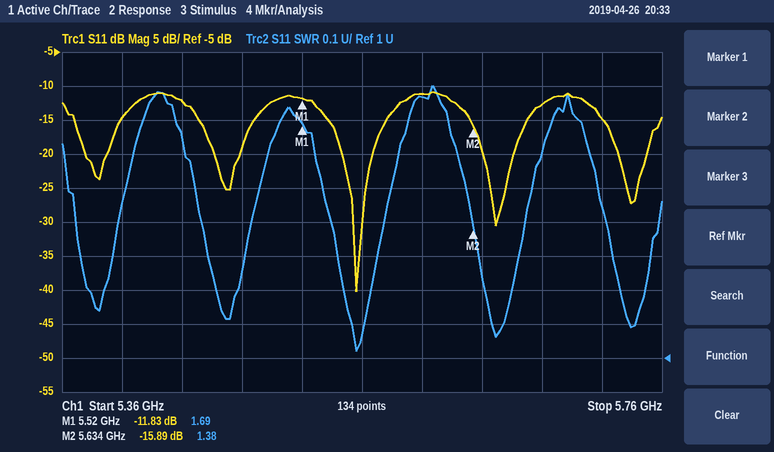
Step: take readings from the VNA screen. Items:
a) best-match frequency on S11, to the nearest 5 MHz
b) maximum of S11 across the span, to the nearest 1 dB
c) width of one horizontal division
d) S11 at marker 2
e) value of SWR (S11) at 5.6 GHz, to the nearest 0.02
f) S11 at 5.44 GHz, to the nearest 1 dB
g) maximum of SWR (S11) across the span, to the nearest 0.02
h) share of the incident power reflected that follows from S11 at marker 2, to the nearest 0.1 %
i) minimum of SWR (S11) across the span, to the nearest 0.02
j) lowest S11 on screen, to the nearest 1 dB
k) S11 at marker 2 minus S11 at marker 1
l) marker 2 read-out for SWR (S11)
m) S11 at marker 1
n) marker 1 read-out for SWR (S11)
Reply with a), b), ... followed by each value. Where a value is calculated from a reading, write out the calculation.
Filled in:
a) 5.555 GHz
b) -11 dB
c) 40 MHz
d) -15.89 dB
e) 1.76
f) -12 dB
g) 1.80
h) 10^(-15.89/10) ≈ 2.6 %
i) 1.02
j) -40 dB
k) -15.89 − (-11.83) = -4.06 dB
l) 1.38
m) -11.83 dB
n) 1.69
